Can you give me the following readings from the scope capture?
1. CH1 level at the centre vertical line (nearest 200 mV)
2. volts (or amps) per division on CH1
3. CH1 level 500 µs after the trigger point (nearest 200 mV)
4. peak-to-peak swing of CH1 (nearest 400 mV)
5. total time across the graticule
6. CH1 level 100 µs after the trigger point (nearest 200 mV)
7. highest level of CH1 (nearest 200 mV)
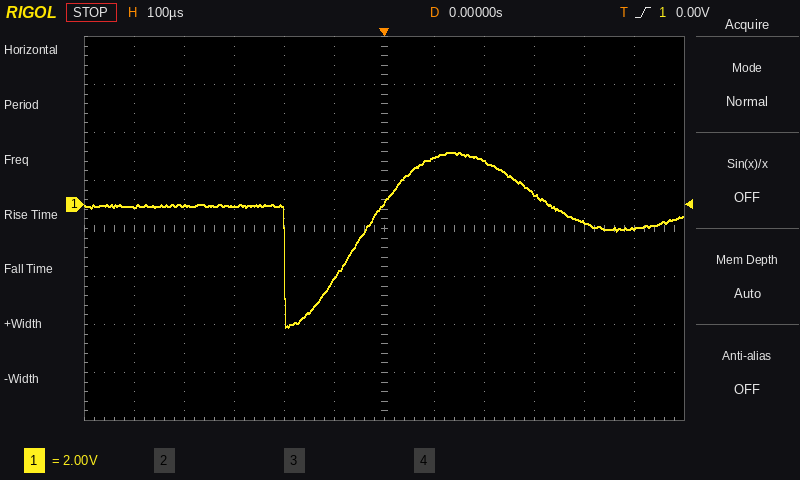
0.0 V
2 V
-1.0 V
7.2 V
1.2 ms
2.0 V
2.2 V
